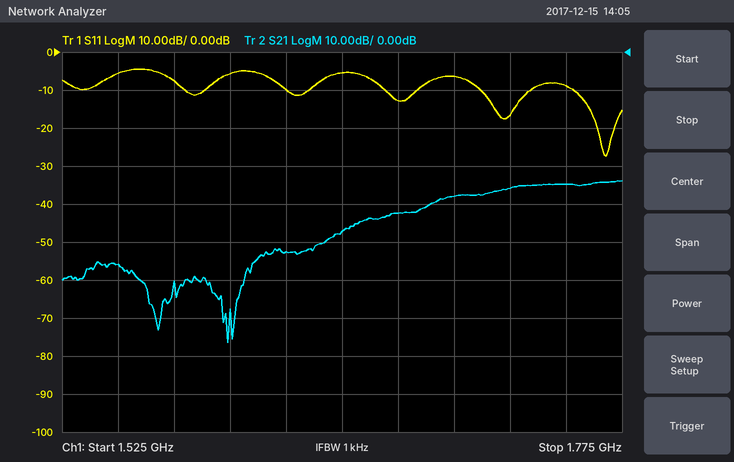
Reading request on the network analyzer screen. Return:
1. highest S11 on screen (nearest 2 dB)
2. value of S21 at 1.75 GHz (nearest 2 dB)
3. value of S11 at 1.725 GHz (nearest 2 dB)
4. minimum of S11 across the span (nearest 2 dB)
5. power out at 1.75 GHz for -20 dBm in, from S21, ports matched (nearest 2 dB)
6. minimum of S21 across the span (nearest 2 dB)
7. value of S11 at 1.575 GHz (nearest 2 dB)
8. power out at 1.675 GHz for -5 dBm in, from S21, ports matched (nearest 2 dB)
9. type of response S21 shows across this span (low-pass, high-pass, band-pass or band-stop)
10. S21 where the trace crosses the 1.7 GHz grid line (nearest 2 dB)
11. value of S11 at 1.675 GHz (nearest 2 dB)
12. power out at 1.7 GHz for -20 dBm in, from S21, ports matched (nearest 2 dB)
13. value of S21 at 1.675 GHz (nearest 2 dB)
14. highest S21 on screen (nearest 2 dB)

-4 dB
-34 dB
-16 dB
-28 dB
-54 dBm
-76 dB
-8 dB
-48 dBm
high-pass
-38 dB
-12 dB
-58 dBm
-42 dB
-34 dB
